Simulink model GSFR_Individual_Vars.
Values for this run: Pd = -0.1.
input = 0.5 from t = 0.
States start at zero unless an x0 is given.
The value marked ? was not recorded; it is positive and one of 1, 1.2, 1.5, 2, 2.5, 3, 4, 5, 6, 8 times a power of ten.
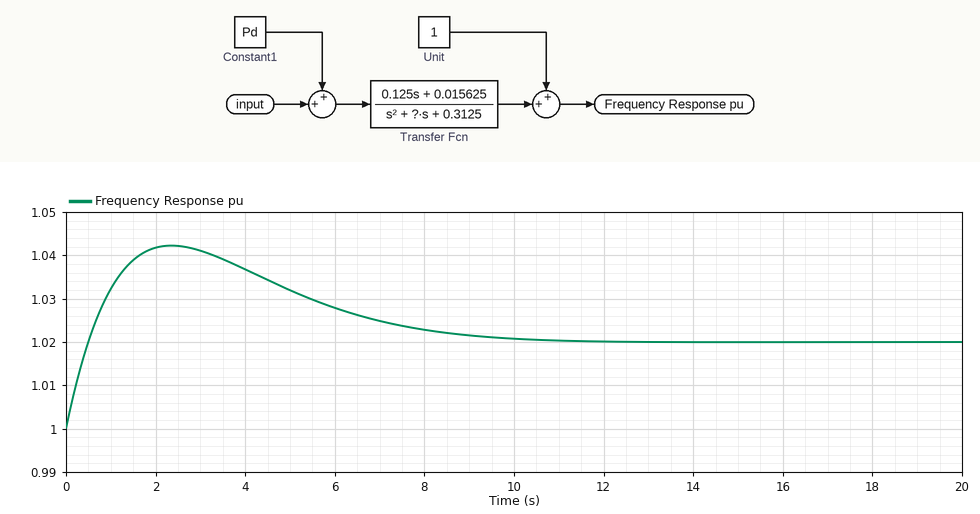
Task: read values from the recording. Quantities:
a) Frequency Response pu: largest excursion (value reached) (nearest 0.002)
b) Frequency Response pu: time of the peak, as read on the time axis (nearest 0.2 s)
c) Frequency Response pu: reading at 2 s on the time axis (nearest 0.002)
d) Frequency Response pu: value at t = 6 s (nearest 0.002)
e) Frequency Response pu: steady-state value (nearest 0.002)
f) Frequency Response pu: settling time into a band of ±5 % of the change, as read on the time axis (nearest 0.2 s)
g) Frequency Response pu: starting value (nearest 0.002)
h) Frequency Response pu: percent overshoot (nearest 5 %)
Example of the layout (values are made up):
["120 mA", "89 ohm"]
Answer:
["1.042", "2.4 s", "1.042", "1.028", "1.020", "9.6 s", "1.000", "110 %"]
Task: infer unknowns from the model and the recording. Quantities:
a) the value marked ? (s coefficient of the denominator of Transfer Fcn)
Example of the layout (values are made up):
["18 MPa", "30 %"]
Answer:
["1"]
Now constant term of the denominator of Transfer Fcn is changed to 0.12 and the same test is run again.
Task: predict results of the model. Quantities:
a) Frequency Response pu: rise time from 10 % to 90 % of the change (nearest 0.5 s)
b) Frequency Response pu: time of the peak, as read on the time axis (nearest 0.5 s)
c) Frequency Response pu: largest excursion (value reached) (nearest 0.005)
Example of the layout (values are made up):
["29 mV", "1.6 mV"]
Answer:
["2.0 s", "5.5 s", "1.055"]
